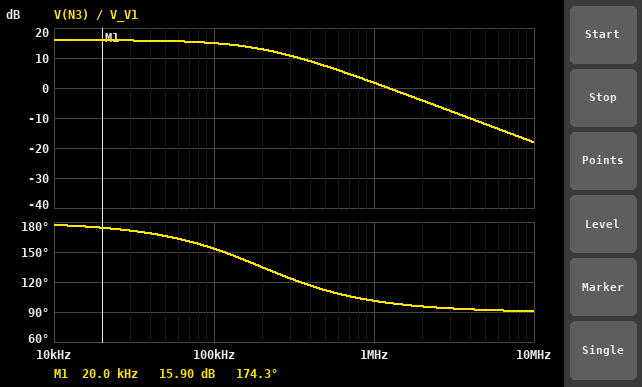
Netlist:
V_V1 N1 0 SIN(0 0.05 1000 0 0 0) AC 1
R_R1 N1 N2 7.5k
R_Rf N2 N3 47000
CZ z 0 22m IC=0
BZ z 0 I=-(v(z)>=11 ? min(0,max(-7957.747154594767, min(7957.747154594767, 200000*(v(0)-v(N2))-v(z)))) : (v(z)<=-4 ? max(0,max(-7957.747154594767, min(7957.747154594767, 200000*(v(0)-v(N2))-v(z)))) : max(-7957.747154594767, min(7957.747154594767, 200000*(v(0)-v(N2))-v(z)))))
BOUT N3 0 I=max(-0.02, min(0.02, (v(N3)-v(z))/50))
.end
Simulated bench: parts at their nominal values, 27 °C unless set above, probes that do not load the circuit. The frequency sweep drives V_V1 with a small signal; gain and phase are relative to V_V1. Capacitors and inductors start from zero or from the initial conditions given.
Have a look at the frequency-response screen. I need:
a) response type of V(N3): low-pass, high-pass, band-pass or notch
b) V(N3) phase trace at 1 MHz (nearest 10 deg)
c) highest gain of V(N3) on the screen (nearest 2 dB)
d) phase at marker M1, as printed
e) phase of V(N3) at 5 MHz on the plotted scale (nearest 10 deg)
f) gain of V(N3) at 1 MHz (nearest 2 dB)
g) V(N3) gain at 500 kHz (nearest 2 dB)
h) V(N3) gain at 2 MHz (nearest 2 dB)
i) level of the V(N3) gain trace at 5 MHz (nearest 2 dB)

low-pass
100 deg
16 dB
174.3 deg
90 deg
2 dB
8 dB
-4 dB
-12 dB
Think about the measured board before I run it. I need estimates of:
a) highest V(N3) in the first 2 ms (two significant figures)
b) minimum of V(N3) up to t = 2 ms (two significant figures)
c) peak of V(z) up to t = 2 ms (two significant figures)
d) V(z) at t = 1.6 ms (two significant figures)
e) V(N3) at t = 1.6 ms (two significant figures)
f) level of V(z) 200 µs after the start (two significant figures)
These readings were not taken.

310 mV
-310 mV
310 mV
180 mV
180 mV
-300 mV
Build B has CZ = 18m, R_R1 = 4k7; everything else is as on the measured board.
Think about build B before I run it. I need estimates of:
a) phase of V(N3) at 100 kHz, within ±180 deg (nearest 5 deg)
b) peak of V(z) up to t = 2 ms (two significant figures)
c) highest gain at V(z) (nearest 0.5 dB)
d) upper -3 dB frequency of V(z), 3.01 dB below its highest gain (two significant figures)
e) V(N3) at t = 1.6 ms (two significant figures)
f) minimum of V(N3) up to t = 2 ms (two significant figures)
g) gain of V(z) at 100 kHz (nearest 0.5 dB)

150 deg
500 mV
20.0 dB
160 kHz
290 mV
-500 mV
18.5 dB
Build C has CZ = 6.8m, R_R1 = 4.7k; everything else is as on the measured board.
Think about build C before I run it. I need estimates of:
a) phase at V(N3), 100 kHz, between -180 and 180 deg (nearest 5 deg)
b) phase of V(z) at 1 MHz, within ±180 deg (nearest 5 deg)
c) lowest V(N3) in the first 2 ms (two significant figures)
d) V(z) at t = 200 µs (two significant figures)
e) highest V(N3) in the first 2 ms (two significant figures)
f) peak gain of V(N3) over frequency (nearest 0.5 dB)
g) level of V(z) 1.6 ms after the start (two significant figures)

165 deg
115 deg
-500 mV
-480 mV
500 mV
20.0 dB
290 mV
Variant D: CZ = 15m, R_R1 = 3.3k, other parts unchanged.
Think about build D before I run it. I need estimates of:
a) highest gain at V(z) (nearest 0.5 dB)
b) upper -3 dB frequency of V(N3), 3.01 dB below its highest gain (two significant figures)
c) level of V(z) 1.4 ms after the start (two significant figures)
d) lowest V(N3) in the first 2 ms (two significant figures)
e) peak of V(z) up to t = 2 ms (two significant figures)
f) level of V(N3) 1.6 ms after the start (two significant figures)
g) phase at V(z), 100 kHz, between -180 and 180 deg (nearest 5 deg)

23.0 dB
140 kHz
-420 mV
-710 mV
710 mV
410 mV
145 deg
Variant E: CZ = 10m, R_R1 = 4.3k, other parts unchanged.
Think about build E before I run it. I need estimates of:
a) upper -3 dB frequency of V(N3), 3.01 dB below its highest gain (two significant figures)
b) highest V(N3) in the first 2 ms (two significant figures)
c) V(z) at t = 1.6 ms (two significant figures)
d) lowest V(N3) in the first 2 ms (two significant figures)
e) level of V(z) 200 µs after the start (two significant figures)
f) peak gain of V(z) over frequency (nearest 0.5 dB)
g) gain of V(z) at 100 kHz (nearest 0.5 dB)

270 kHz
550 mV
320 mV
-550 mV
-520 mV
21.0 dB
20.0 dB
